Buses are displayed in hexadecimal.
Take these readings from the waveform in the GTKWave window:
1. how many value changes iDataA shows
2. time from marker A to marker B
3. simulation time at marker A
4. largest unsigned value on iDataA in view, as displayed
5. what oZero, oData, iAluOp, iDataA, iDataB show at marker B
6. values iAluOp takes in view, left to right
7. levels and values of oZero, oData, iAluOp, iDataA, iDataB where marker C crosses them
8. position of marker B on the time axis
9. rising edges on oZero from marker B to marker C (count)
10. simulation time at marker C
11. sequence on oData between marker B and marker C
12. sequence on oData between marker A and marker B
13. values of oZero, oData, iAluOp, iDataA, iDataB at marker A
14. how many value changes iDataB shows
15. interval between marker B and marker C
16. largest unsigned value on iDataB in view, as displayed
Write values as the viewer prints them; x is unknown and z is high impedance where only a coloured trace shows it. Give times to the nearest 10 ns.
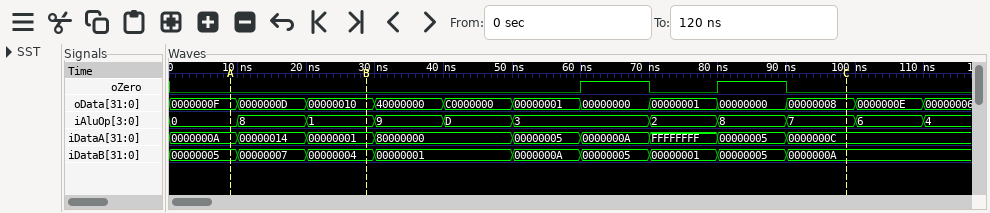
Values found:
8
20 ns
10 ns
FFFFFFFF
oZero=0, oData=00000010, iAluOp=1, iDataA=00000001, iDataB=00000004
0, 8, 1, 9, D, 3, 2, 8, 7, 6, 4
oZero=0, oData=00000008, iAluOp=7, iDataA=0000000C, iDataB=0000000A
30 ns
2
100 ns
00000010, 40000000, C0000000, 00000001, 00000000, 00000001, 00000000, 00000008
0000000F, 0000000D, 00000010
oZero=0, oData=0000000F, iAluOp=0, iDataA=0000000A, iDataB=00000005
8
70 ns
0000000A
